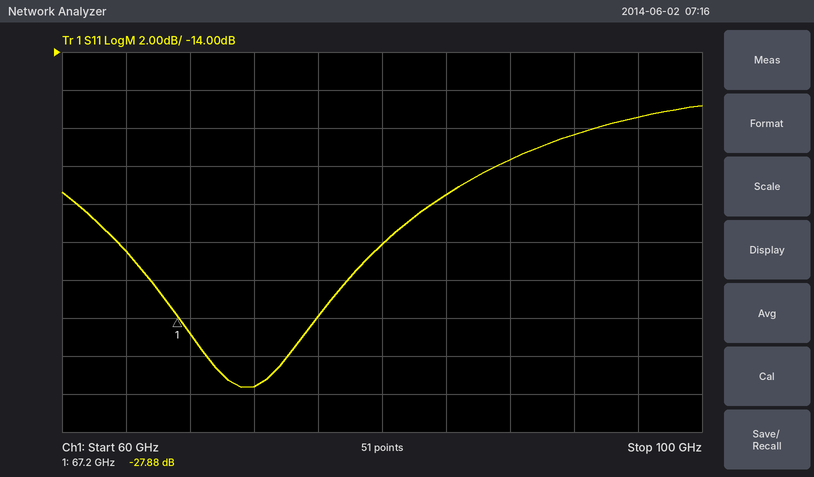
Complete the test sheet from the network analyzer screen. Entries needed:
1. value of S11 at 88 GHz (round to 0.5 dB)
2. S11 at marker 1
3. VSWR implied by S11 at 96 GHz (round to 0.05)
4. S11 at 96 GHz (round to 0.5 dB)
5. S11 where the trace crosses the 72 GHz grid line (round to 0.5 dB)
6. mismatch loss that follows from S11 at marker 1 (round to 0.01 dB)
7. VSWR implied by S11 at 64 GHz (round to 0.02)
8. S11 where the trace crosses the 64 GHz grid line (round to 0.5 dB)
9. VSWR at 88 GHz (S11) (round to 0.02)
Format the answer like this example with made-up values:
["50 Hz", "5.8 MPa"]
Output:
["-19.5 dB", "-27.88 dB", "1.30", "-17.5 dB", "-31.5 dB", "0.01 dB", "1.12", "-24.5 dB", "1.24"]
